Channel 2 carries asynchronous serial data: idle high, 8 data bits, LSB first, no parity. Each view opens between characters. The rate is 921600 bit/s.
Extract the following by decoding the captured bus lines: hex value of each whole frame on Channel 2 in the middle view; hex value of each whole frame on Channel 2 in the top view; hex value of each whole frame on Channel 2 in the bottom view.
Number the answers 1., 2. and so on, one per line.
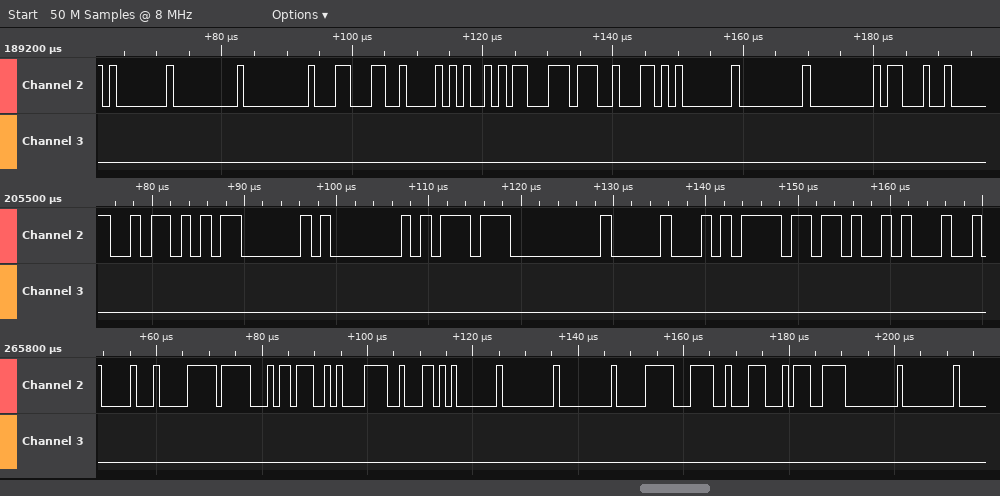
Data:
1. 5A, 03, 01, DD, 00, 10, BD, 4B
2. 01, 00, 00, 8C, 42, A9, DC, 62, 01, 00, 00, 23
3. 10, F0, 1F, 3B, E1, 62, 01, 00, 00, F0, 3C, 1C, E7, 00, 00
